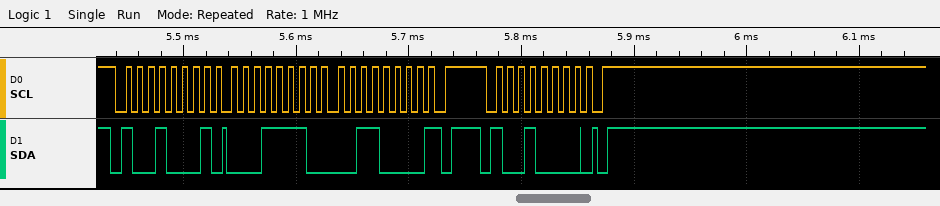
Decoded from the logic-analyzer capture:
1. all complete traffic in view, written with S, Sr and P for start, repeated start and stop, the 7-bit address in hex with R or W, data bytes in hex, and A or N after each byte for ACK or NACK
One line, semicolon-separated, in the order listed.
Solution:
S 48R A 1E A 30 N P S 48W A P
